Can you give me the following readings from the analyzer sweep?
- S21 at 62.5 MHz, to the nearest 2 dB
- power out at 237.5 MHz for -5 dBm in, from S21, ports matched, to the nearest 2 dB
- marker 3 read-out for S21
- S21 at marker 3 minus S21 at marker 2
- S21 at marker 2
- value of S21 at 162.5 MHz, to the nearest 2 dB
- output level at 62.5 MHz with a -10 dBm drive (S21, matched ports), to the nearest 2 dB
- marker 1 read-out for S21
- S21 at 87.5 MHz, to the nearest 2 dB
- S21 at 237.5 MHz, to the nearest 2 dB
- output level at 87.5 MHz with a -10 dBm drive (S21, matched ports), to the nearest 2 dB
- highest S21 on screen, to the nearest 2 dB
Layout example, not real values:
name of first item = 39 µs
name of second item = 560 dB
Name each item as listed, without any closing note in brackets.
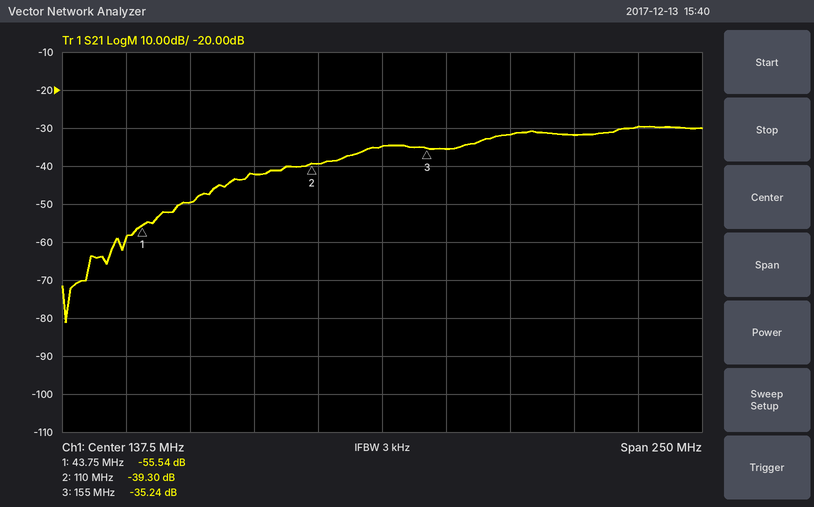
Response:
S21 at 62.5 MHz, to the nearest 2 dB = -50 dB
power out at 237.5 MHz for -5 dBm in, from S21, ports matched, to the nearest 2 dB = -34 dBm
marker 3 read-out for S21 = -35.24 dB
S21 at marker 3 minus S21 at marker 2 = 4.06 dB
S21 at marker 2 = -39.30 dB
value of S21 at 162.5 MHz, to the nearest 2 dB = -36 dB
output level at 62.5 MHz with a -10 dBm drive (S21, matched ports), to the nearest 2 dB = -60 dBm
marker 1 read-out for S21 = -55.54 dB
S21 at 87.5 MHz, to the nearest 2 dB = -42 dB
S21 at 237.5 MHz, to the nearest 2 dB = -30 dB
output level at 87.5 MHz with a -10 dBm drive (S21, matched ports), to the nearest 2 dB = -52 dBm
highest S21 on screen, to the nearest 2 dB = -30 dB
